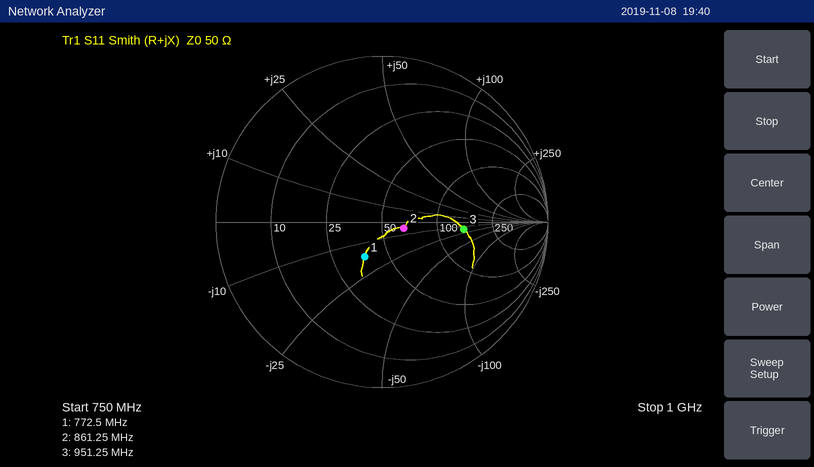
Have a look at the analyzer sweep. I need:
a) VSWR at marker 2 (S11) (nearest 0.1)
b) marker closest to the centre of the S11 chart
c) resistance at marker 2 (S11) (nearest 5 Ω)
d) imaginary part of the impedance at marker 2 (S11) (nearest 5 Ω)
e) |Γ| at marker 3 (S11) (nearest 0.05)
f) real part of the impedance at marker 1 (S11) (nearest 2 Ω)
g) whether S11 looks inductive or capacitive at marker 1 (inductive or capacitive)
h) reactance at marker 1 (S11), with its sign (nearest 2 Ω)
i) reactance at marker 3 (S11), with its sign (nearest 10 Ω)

1.3
marker 2
65 Ω
-5 Ω
0.50
38 Ω
capacitive
-16 Ω
-20 Ω
